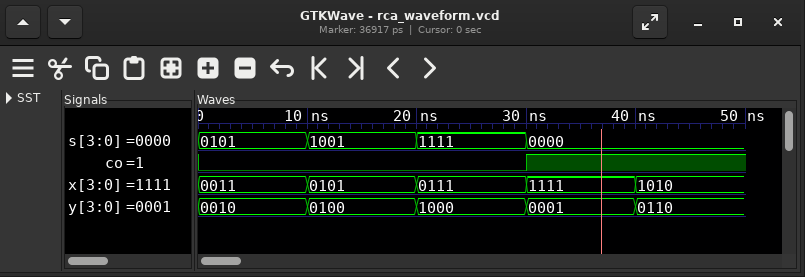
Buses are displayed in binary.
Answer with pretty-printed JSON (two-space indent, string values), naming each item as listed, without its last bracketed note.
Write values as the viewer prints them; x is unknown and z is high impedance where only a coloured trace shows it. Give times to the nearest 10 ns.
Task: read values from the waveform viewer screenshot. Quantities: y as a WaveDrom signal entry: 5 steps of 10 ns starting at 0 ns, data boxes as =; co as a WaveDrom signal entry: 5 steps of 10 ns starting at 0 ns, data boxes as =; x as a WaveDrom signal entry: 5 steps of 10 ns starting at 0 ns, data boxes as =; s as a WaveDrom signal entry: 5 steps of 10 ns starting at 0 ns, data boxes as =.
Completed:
{
  "y as a WaveDrom signal entry: 5 steps of 10 ns starting at 0 ns, data boxes as =": "{name: 'y', wave: '=====', data: '0010 0100 1000 0001 0110'}",
  "co as a WaveDrom signal entry: 5 steps of 10 ns starting at 0 ns, data boxes as =": "{name: 'co', wave: '0..1.'}",
  "x as a WaveDrom signal entry: 5 steps of 10 ns starting at 0 ns, data boxes as =": "{name: 'x', wave: '=====', data: '0011 0101 0111 1111 1010'}",
  "s as a WaveDrom signal entry: 5 steps of 10 ns starting at 0 ns, data boxes as =": "{name: 's', wave: '====.', data: '0101 1001 1111 0000'}"
}
